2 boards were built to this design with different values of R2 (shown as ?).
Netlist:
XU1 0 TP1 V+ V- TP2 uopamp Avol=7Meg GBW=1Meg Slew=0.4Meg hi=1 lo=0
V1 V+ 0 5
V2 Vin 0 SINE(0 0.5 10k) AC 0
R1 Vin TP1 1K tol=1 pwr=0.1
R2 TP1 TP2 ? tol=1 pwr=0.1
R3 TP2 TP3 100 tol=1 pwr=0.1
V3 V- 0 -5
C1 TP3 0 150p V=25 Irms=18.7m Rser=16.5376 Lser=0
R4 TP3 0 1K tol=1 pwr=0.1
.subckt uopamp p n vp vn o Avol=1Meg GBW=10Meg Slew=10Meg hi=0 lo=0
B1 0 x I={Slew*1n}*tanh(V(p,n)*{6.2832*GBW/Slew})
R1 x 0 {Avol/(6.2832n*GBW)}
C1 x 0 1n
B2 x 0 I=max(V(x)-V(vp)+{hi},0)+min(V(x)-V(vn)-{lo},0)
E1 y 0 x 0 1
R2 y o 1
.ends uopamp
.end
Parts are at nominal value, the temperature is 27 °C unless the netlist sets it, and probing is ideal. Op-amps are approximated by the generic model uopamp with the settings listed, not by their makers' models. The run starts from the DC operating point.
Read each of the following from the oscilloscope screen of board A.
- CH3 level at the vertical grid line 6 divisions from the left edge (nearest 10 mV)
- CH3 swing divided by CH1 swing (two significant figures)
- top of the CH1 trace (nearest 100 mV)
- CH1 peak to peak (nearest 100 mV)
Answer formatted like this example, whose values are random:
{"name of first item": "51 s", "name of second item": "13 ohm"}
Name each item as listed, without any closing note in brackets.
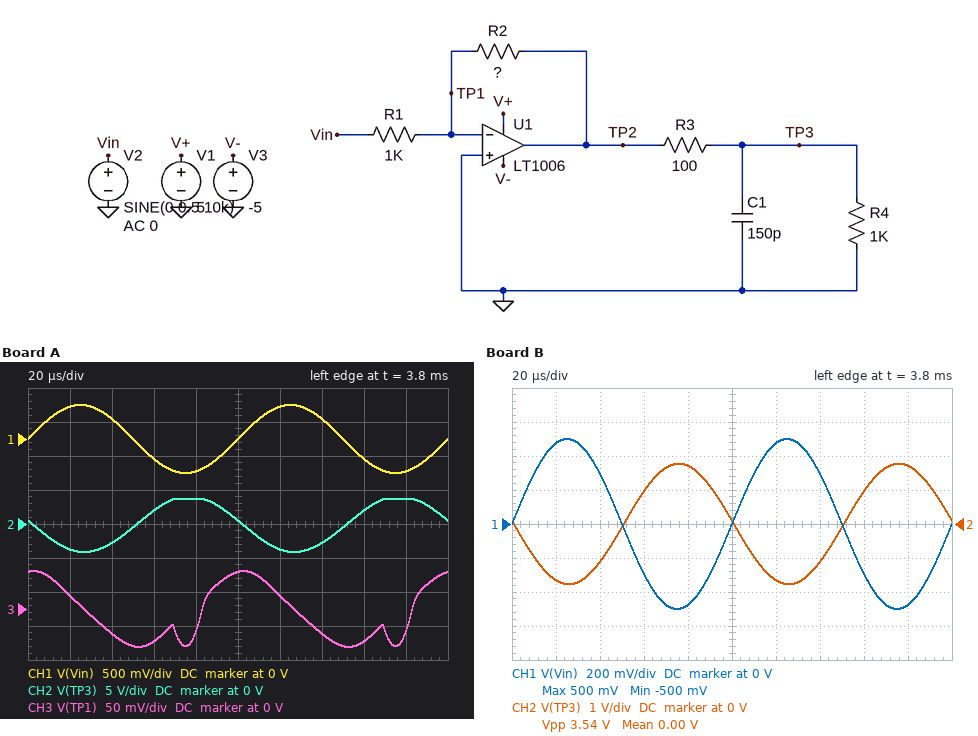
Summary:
{"CH3 level at the vertical grid line 6 divisions from the left edge": "20 mV", "CH3 swing divided by CH1 swing": "0.11", "top of the CH1 trace": "500 mV", "CH1 peak to peak": "1.0 V"}
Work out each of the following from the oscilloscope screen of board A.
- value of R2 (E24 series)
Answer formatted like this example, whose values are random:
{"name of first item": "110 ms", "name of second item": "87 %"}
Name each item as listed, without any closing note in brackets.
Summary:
{"value of R2": "9.1 kΩ"}
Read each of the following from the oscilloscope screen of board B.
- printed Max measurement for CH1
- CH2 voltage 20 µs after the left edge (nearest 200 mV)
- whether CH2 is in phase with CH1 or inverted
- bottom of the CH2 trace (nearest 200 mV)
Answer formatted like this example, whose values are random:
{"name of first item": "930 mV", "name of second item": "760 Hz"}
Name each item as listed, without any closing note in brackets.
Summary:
{"printed Max measurement for CH1": "500 mV", "CH2 voltage 20 µs after the left edge": "-1.6 V", "whether CH2 is in phase with CH1 or inverted": "inverted", "bottom of the CH2 trace": "-1.8 V"}
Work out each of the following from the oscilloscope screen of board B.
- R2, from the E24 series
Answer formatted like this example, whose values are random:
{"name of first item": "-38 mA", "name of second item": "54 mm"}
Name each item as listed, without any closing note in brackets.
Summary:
{"R2, from the E24 series": "3.9 kΩ"}
